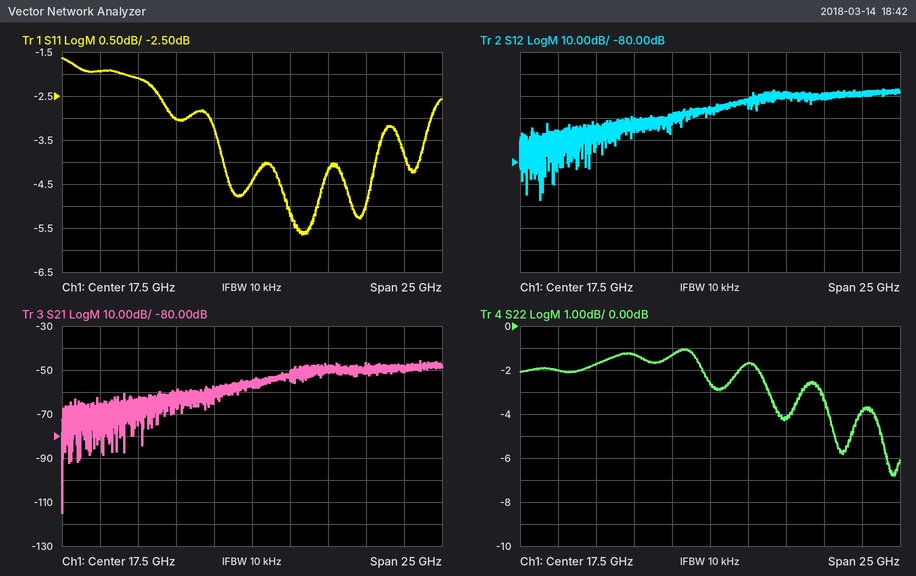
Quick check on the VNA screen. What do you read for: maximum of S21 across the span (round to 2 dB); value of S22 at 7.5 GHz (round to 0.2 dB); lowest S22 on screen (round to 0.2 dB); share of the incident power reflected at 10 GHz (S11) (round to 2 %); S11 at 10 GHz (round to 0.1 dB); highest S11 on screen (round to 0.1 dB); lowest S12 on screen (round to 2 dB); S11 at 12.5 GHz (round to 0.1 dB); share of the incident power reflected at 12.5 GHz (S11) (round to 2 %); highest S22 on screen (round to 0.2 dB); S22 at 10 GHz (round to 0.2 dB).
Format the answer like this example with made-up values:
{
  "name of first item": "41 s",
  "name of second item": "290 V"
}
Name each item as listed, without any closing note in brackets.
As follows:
{
  "maximum of S21 across the span": "-46 dB",
  "value of S22 at 7.5 GHz": "-2.0 dB",
  "lowest S22 on screen": "-6.8 dB",
  "share of the incident power reflected at 10 GHz (S11)": "62 %",
  "S11 at 10 GHz": "-2.1 dB",
  "highest S11 on screen": "-1.6 dB",
  "lowest S12 on screen": "-98 dB",
  "S11 at 12.5 GHz": "-3.0 dB",
  "share of the incident power reflected at 12.5 GHz (S11)": "50 %",
  "highest S22 on screen": "-1.0 dB",
  "S22 at 10 GHz": "-1.8 dB"
}
